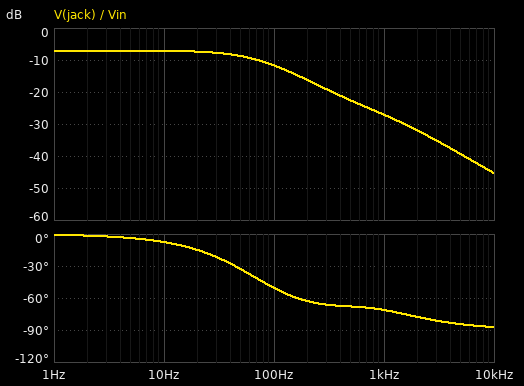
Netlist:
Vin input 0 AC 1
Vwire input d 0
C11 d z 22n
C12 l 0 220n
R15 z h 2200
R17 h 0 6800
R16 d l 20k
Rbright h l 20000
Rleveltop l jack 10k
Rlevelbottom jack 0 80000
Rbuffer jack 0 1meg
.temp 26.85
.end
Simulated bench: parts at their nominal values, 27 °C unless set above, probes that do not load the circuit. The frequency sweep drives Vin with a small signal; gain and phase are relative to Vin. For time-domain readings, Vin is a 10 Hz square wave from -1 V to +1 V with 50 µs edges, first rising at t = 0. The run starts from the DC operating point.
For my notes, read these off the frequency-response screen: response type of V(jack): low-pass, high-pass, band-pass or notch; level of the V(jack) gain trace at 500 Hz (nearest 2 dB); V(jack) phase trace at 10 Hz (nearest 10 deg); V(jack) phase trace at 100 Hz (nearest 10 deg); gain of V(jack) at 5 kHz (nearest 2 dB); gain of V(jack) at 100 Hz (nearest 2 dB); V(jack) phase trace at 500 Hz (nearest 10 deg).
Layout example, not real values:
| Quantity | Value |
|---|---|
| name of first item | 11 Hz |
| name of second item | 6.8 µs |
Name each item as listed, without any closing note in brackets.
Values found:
| Quantity | Value |
|---|---|
| response type of V(jack): low-pass, high-pass, band-pass or notch | low-pass |
| level of the V(jack) gain trace at 500 Hz | -22 dB |
| V(jack) phase trace at 10 Hz | -10 deg |
| V(jack) phase trace at 100 Hz | -50 deg |
| gain of V(jack) at 5 kHz | -40 dB |
| gain of V(jack) at 100 Hz | -12 dB |
| V(jack) phase trace at 500 Hz | -70 deg |
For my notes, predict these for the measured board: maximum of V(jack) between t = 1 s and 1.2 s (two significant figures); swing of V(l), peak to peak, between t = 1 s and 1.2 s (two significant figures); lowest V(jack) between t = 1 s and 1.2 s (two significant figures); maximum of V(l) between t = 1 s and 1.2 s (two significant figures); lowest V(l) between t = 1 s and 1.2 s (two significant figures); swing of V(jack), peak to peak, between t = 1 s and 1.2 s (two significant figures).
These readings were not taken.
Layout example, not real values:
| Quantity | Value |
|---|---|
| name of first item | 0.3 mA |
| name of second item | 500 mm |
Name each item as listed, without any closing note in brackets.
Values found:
| Quantity | Value |
|---|---|
| maximum of V(jack) between t = 1 s and 1.2 s | 440 mV |
| swing of V(l), peak to peak, between t = 1 s and 1.2 s | 1.0 V |
| lowest V(jack) between t = 1 s and 1.2 s | -440 mV |
| maximum of V(l) between t = 1 s and 1.2 s | 500 mV |
| lowest V(l) between t = 1 s and 1.2 s | -500 mV |
| swing of V(jack), peak to peak, between t = 1 s and 1.2 s | 890 mV |
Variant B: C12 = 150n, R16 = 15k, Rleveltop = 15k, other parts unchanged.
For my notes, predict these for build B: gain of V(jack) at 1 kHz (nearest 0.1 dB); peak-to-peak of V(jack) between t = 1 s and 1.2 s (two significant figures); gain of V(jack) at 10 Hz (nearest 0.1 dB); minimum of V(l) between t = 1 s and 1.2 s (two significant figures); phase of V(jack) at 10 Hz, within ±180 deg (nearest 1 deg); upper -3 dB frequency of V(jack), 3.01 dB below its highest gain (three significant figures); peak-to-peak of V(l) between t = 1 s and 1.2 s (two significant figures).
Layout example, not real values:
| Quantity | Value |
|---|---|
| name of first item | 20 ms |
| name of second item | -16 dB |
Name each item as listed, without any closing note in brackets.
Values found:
| Quantity | Value |
|---|---|
| gain of V(jack) at 1 kHz | -22.5 dB |
| peak-to-peak of V(jack) between t = 1 s and 1.2 s | 960 mV |
| gain of V(jack) at 10 Hz | -6.4 dB |
| minimum of V(l) between t = 1 s and 1.2 s | -580 mV |
| phase of V(jack) at 10 Hz, within ±180 deg | -4 deg |
| upper -3 dB frequency of V(jack), 3.01 dB below its highest gain | 123 Hz |
| peak-to-peak of V(l) between t = 1 s and 1.2 s | 1.2 V |
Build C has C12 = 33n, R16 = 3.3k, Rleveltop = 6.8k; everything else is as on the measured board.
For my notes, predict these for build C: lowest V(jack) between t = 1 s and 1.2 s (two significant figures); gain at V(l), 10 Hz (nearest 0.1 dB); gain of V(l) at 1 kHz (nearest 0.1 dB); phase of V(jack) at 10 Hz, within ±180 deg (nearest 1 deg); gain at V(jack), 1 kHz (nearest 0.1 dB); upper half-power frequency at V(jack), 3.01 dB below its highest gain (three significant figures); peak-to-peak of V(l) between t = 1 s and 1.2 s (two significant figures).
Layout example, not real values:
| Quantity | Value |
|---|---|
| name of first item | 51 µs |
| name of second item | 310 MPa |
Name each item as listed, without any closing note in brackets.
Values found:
| Quantity | Value |
|---|---|
| lowest V(jack) between t = 1 s and 1.2 s | -790 mV |
| gain at V(l), 10 Hz | -1.3 dB |
| gain of V(l) at 1 kHz | -2.2 dB |
| phase of V(jack) at 10 Hz, within ±180 deg | 0 deg |
| gain at V(jack), 1 kHz | -3.0 dB |
| upper half-power frequency at V(jack), 3.01 dB below its highest gain | 1.96 kHz |
| peak-to-peak of V(l) between t = 1 s and 1.2 s | 1.7 V |
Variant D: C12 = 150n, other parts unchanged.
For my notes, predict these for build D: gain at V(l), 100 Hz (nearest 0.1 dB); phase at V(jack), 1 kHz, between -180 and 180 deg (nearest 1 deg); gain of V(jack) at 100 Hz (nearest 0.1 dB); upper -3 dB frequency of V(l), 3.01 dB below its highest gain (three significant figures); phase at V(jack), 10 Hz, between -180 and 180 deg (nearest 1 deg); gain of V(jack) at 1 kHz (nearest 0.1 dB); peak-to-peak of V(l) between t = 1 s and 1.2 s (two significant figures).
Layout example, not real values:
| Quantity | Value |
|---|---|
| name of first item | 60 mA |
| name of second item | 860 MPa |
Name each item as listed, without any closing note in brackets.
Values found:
| Quantity | Value |
|---|---|
| gain at V(l), 100 Hz | -8.7 dB |
| phase at V(jack), 1 kHz, between -180 and 180 deg | -69 deg |
| gain of V(jack) at 100 Hz | -9.8 dB |
| upper -3 dB frequency of V(l), 3.01 dB below its highest gain | 106 Hz |
| phase at V(jack), 10 Hz, between -180 and 180 deg | -5 deg |
| gain of V(jack) at 1 kHz | -23.8 dB |
| peak-to-peak of V(l) between t = 1 s and 1.2 s | 1.0 V |
